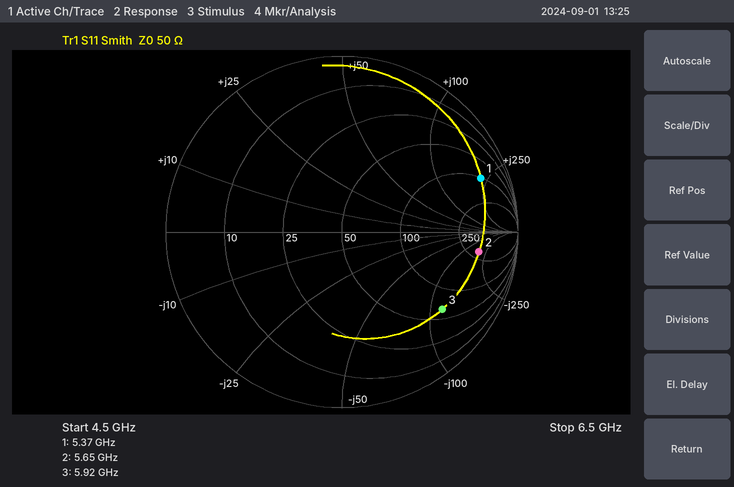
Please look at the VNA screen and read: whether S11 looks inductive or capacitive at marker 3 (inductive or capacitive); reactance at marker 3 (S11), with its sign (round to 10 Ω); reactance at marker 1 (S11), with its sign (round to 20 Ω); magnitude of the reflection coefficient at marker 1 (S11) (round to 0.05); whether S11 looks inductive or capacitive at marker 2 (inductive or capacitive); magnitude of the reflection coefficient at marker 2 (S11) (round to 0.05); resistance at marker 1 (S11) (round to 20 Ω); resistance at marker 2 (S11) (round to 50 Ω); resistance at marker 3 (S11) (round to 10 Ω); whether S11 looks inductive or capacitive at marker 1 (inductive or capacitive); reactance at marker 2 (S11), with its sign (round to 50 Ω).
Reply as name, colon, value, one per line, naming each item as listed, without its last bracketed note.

whether S11 looks inductive or capacitive at marker 3: capacitive
reactance at marker 3 (S11), with its sign: -120 Ω
reactance at marker 1 (S11), with its sign: +220 Ω
magnitude of the reflection coefficient at marker 1 (S11): 0.85
whether S11 looks inductive or capacitive at marker 2: capacitive
magnitude of the reflection coefficient at marker 2 (S11): 0.80
resistance at marker 1 (S11): 100 Ω
resistance at marker 2 (S11): 300 Ω
resistance at marker 3 (S11): 60 Ω
whether S11 looks inductive or capacitive at marker 1: inductive
reactance at marker 2 (S11), with its sign: -200 Ω
